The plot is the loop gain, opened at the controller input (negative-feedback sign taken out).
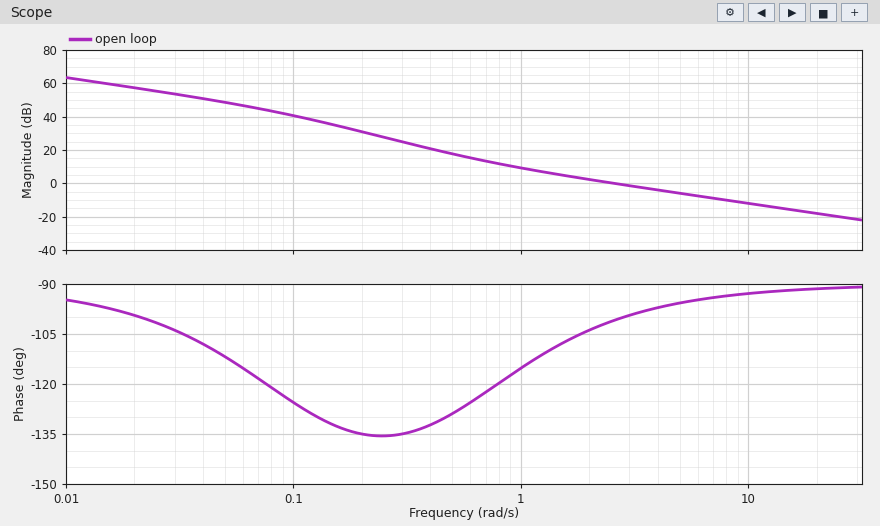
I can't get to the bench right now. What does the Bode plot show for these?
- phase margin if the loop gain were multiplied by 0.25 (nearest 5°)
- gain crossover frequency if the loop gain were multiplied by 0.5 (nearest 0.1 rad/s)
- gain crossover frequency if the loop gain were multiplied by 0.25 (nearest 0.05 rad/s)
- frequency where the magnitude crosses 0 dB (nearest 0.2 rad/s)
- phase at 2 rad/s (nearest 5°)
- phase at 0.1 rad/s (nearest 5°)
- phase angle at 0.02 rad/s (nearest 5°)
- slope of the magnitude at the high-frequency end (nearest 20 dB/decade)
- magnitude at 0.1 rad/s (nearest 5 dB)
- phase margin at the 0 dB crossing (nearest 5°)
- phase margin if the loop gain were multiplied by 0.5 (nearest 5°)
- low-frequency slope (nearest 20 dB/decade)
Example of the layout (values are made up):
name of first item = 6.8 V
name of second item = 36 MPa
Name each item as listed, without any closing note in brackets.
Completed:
phase margin if the loop gain were multiplied by 0.25 = 60°
gain crossover frequency if the loop gain were multiplied by 0.5 = 1.4 rad/s
gain crossover frequency if the loop gain were multiplied by 0.25 = 0.80 rad/s
frequency where the magnitude crosses 0 dB = 2.6 rad/s
phase at 2 rad/s = -105°
phase at 0.1 rad/s = -125°
phase angle at 0.02 rad/s = -100°
slope of the magnitude at the high-frequency end = -20 dB/decade
magnitude at 0.1 rad/s = 40 dB
phase margin at the 0 dB crossing = 80°
phase margin if the loop gain were multiplied by 0.5 = 70°
low-frequency slope = -20 dB/decade
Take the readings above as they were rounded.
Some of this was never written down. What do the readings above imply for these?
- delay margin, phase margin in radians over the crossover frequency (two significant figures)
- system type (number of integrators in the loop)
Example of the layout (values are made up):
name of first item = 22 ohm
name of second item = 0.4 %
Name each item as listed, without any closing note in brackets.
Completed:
delay margin, phase margin in radians over the crossover frequency = 0.54 s
system type = 1
